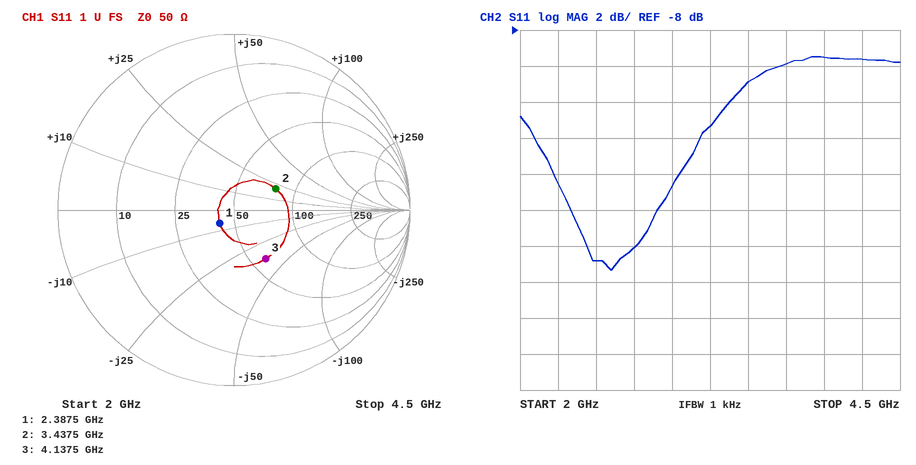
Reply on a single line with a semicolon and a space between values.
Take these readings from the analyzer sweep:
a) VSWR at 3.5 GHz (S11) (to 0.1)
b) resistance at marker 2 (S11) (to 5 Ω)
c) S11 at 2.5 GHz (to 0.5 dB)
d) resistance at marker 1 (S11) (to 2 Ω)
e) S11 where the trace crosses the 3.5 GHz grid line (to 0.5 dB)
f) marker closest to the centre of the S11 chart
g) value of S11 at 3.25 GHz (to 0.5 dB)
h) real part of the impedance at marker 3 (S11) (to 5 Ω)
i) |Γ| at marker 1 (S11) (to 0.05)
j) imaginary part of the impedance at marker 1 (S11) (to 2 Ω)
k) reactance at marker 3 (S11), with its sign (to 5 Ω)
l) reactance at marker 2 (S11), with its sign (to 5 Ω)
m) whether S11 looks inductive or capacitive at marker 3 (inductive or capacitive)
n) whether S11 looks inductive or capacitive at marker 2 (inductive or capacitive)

1.8; 80 Ω; -21.0 dB; 42 Ω; -11.0 dB; marker 1; -13.5 dB; 60 Ω; 0.10; -6 Ω; -35 Ω; +20 Ω; capacitive; inductive
